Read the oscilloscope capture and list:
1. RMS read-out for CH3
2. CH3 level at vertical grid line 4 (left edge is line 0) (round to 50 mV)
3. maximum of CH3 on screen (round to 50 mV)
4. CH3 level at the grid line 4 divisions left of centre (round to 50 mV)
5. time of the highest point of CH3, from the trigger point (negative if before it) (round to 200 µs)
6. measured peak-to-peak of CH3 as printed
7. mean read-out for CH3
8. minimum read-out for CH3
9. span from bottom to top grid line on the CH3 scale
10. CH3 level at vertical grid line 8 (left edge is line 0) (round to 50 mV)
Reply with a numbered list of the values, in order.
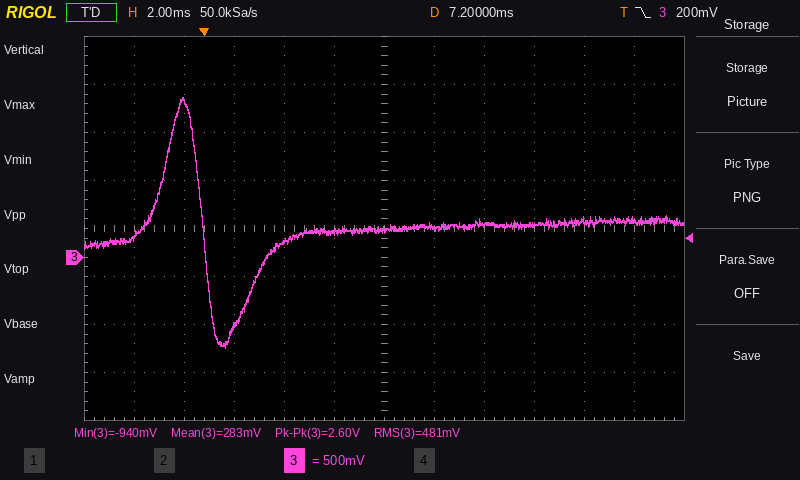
1. 481 mV
2. 150 mV
3. 1.65 V
4. 1.60 V
5. -800 µs
6. 2.60 V
7. 283 mV
8. -940 mV
9. 4 V
10. 350 mV
